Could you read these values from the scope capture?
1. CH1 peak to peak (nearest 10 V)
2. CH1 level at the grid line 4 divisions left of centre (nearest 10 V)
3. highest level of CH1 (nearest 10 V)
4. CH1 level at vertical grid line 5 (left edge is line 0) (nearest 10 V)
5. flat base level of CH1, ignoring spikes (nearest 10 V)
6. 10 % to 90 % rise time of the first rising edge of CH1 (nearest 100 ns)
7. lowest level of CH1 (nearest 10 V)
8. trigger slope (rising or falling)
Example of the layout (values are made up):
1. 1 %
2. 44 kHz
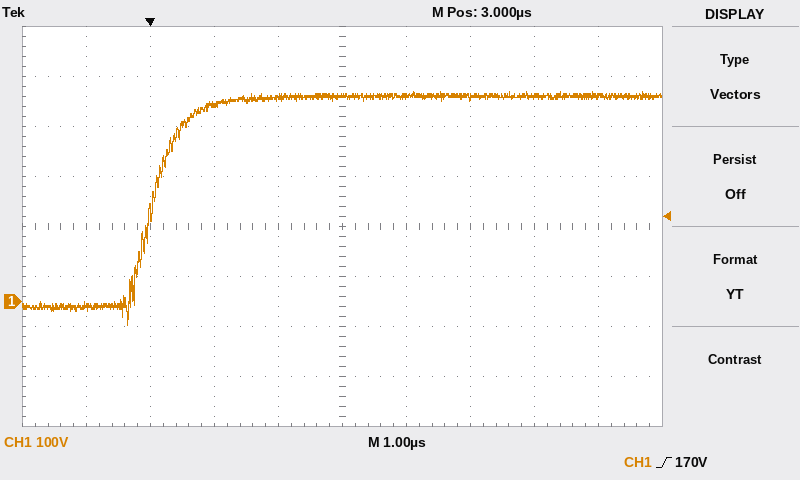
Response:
1. 470 V
2. -10 V
3. 420 V
4. 410 V
5. -10 V
6. 900 ns
7. -50 V
8. rising
